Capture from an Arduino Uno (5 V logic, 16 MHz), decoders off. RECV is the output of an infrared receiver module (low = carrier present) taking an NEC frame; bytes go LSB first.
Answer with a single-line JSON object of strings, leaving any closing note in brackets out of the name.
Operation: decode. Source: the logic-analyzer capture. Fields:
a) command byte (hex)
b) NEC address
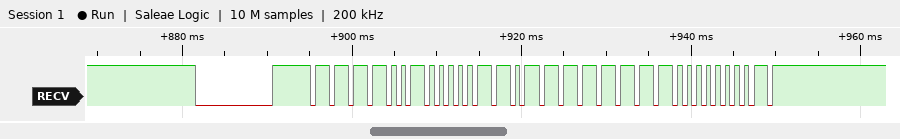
{"command byte": "0x7F", "NEC address": "0x4F"}
